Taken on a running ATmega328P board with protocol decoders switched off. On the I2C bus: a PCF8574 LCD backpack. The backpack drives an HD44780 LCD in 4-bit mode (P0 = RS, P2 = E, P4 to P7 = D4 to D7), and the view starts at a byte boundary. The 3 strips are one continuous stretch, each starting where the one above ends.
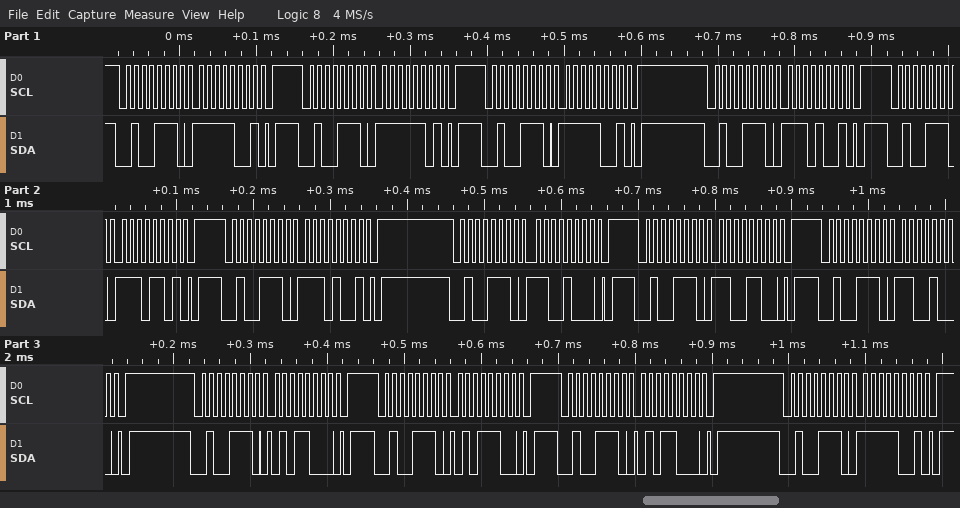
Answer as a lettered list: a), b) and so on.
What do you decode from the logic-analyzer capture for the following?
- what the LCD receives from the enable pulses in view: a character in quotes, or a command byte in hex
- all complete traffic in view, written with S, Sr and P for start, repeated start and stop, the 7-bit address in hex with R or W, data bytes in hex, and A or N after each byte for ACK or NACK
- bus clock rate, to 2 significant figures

a) data 0xFE 0xC5
b) S 27W A F9 A P S 27W A FD A P S 27W A F9 A P S 27W A E9 A P S 27W A ED A P S 27W A E9 A P S 27W A C8 A P S 27W A CC A P S 27W A C8 A P S 27W A 58 A P S 27W A 5C A P S 27W A 58 A P S 27W A F9 A P
c) 100 kHz
